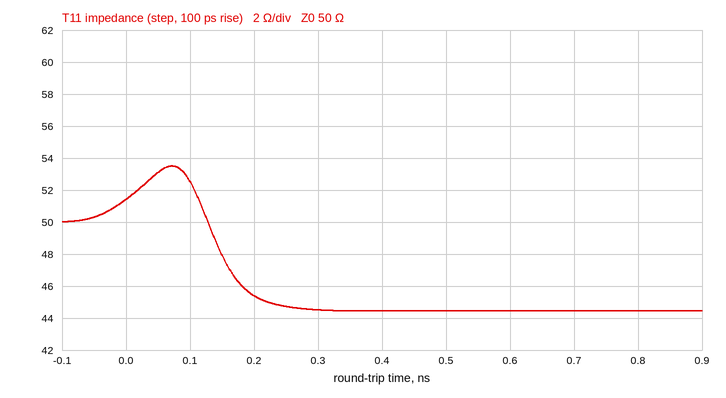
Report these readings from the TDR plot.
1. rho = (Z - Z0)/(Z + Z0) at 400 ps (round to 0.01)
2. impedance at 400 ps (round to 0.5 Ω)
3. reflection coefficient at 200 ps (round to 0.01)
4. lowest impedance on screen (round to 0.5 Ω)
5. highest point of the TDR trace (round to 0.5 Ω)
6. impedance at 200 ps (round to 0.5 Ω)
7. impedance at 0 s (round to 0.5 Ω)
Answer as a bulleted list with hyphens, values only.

- -0.06
- 44.5 Ω
- -0.05
- 44.5 Ω
- 53.5 Ω
- 45.5 Ω
- 51.5 Ω
